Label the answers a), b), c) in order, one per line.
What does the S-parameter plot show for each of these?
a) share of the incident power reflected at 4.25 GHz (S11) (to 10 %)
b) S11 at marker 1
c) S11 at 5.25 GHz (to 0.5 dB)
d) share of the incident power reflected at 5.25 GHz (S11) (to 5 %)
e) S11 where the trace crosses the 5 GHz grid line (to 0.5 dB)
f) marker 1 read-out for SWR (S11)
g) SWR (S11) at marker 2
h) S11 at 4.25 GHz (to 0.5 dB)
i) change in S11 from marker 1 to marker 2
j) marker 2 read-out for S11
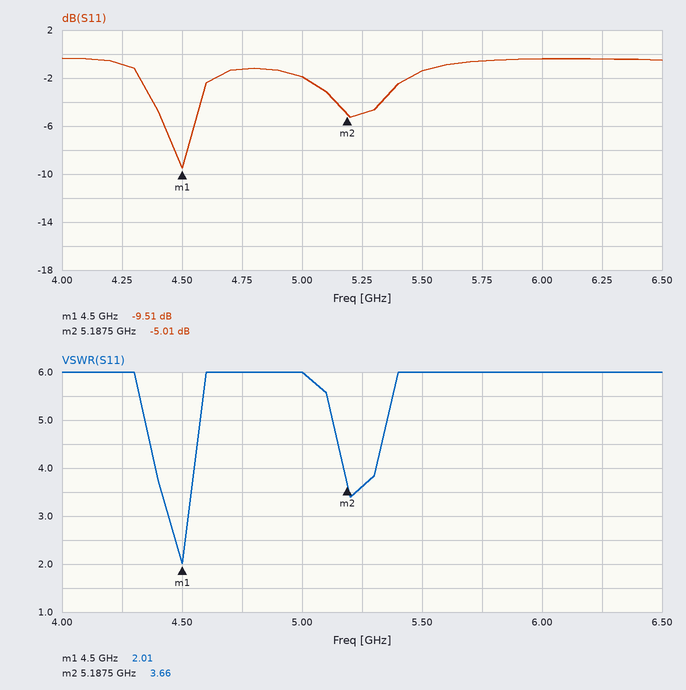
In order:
a) 80 %
b) -9.51 dB
c) -5.0 dB
d) 30 %
e) -2.0 dB
f) 2.01
g) 3.66
h) -1.0 dB
i) 4.50 dB
j) -5.01 dB
